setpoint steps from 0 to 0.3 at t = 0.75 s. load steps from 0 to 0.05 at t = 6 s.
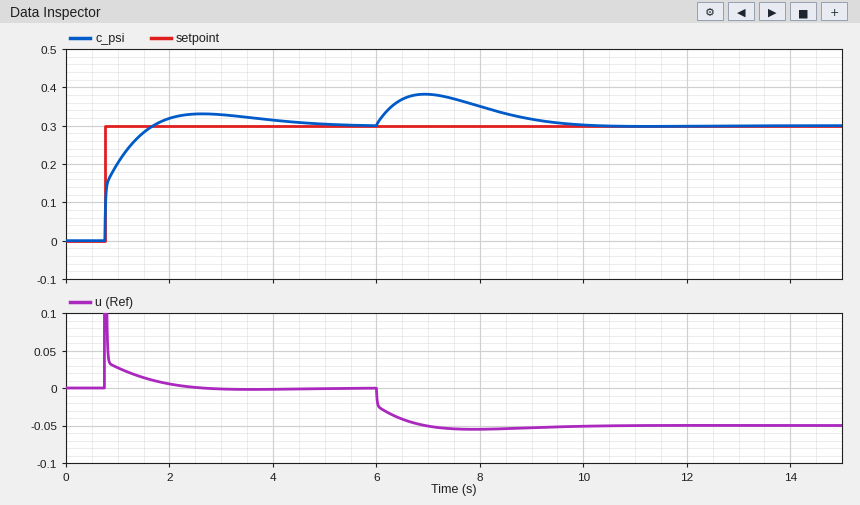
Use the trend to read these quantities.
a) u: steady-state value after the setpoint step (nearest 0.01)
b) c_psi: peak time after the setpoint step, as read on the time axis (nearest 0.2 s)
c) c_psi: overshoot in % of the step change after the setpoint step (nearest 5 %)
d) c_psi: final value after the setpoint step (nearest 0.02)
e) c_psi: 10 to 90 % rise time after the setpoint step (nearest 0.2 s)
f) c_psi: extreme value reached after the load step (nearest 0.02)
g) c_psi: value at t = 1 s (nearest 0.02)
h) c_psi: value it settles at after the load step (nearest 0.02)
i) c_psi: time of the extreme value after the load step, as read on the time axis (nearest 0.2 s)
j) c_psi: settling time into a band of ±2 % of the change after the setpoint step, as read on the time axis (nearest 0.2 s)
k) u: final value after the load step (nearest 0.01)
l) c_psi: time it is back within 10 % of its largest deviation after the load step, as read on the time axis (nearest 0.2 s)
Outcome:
0.00
2.6 s
10 %
0.30
0.6 s
0.38
0.20
0.30
7.0 s
4.8 s
-0.05
9.4 s
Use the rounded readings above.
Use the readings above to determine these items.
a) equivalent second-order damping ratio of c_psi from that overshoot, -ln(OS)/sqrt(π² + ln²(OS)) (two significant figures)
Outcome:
0.59
